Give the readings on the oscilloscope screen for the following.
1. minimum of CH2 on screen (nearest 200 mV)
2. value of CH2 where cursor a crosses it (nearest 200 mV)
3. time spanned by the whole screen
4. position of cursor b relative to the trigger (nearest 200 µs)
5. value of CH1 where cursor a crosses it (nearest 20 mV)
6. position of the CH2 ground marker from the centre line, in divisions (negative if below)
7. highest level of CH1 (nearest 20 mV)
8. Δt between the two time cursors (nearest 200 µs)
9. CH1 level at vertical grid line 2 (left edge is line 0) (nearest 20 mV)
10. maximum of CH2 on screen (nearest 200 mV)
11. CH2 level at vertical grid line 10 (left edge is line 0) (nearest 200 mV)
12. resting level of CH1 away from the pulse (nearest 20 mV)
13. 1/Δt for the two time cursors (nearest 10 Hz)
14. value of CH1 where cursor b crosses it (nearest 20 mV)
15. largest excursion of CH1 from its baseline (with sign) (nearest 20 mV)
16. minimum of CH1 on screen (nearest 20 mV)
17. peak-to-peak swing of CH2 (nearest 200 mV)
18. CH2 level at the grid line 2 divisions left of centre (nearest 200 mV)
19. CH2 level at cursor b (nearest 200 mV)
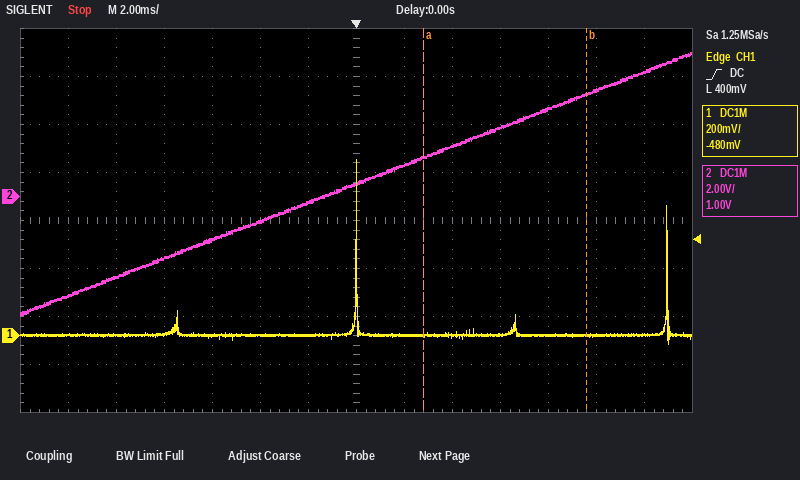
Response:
-5.0 V
1.6 V
28 ms
+9.6 ms
0 mV
+0.5 div
740 mV
6.8 ms
0 mV
6.0 V
2.8 V
0 mV
150 Hz
0 mV
+740 mV
-40 mV
11.0 V
-1.0 V
4.2 V
